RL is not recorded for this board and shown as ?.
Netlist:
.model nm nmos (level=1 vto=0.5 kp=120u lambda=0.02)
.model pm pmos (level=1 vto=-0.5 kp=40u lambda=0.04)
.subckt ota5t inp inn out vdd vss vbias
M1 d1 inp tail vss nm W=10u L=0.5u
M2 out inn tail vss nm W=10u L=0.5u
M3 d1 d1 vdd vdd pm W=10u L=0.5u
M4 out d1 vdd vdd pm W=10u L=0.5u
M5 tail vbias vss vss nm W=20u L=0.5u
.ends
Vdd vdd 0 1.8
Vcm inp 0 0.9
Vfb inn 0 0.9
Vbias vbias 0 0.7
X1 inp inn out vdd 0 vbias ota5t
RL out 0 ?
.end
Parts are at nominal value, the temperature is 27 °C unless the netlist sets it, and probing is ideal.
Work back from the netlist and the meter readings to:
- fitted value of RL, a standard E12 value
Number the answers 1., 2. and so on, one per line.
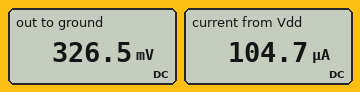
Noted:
1. 39 kΩ
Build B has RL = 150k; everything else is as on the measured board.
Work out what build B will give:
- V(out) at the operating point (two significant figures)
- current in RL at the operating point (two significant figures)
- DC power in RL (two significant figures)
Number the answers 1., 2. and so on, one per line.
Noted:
1. 370 mV
2. 2.5 µA
3. 930 nW
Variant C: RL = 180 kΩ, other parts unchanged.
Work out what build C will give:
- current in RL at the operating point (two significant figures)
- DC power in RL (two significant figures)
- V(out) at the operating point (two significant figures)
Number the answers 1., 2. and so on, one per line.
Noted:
1. 2.1 µA
2. 800 nW
3. 380 mV
